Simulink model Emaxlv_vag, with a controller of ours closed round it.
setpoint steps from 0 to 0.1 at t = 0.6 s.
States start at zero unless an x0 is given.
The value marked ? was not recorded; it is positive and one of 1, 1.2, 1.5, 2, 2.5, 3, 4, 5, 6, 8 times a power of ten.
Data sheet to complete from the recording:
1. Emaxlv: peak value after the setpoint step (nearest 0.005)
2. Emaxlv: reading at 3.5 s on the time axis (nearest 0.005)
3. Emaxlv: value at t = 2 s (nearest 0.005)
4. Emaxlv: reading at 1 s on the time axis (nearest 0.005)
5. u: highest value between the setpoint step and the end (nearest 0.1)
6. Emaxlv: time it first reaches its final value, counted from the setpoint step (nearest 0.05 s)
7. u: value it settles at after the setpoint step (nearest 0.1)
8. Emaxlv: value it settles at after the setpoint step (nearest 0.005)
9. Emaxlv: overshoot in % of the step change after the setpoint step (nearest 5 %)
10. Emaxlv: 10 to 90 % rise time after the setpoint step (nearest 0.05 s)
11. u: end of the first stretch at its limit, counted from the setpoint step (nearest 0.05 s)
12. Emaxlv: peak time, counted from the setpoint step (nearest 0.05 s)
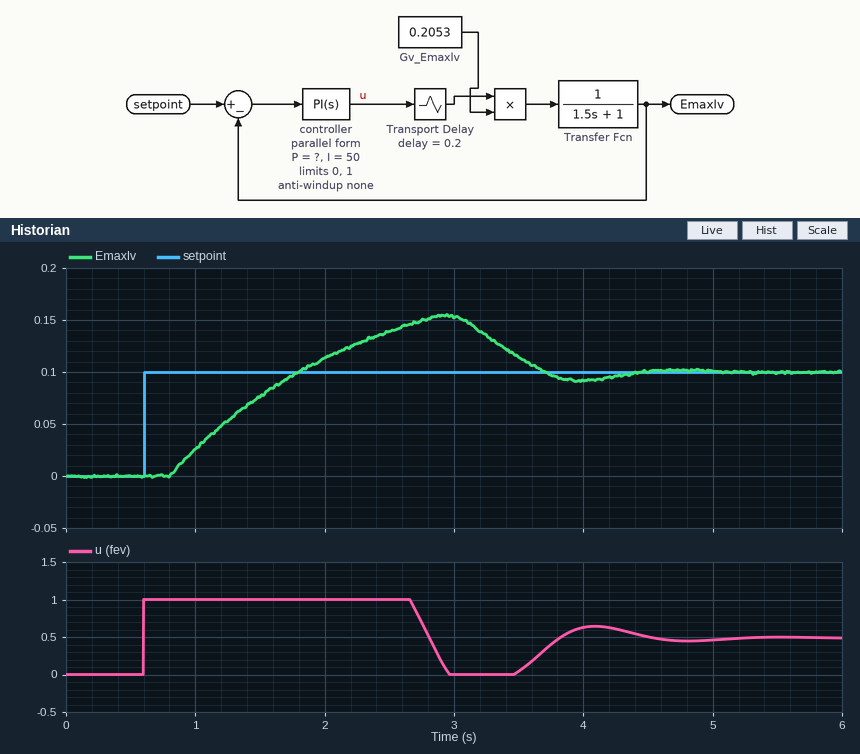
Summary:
0.155
0.115
0.115
0.025
1.0
1.20 s
0.5
0.100
55 %
0.80 s
2.05 s
2.35 s
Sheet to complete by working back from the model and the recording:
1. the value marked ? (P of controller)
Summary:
25
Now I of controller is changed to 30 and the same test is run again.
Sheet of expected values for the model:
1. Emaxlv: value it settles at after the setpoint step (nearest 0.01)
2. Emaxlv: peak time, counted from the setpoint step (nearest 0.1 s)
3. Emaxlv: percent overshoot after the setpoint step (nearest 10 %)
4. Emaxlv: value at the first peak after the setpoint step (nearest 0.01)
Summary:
0.10
2.0 s
40 %
0.14
